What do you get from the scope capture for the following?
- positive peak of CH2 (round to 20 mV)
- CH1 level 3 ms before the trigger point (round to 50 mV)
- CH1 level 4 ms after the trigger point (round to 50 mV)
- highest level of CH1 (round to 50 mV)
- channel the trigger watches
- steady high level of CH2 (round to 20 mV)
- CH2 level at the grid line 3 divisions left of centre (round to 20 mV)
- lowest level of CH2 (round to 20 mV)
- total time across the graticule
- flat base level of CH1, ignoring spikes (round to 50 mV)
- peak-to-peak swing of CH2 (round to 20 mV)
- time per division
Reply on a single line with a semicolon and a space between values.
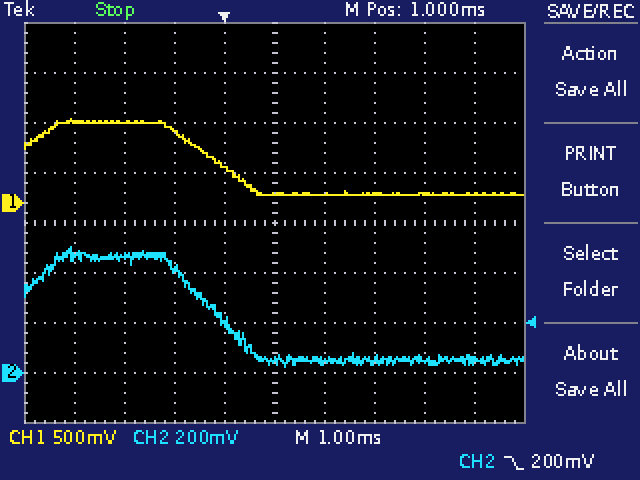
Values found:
500 mV; 800 mV; 100 mV; 850 mV; CH2; 460 mV; 460 mV; 20 mV; 10 ms; 100 mV; 480 mV; 1 ms
